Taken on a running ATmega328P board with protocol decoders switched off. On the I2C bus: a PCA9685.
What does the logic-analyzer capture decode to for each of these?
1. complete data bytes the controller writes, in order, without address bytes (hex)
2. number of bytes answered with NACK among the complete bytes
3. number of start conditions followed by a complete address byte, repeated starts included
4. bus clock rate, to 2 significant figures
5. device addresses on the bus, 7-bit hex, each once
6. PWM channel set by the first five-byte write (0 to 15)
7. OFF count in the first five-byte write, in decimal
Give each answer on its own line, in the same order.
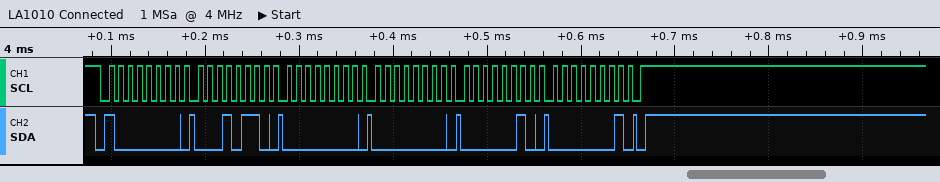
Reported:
16 00 00 02 01
0
1
100 kHz
0x40
4
258
